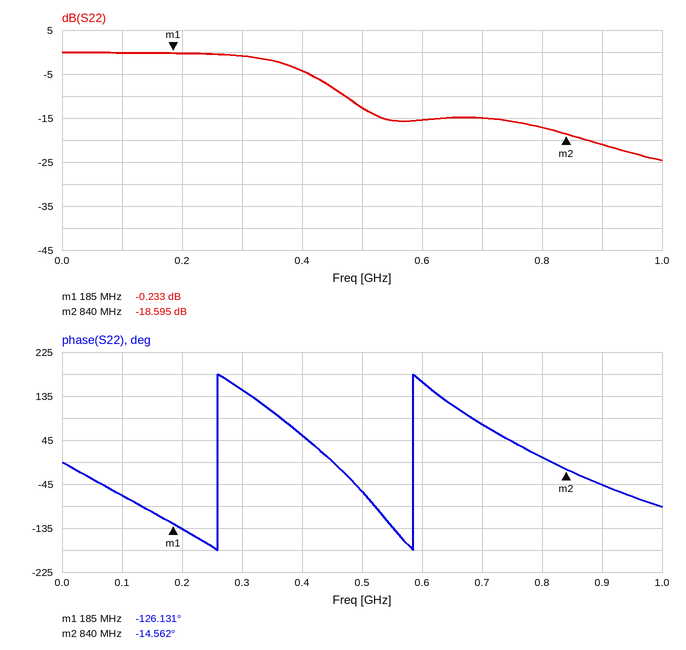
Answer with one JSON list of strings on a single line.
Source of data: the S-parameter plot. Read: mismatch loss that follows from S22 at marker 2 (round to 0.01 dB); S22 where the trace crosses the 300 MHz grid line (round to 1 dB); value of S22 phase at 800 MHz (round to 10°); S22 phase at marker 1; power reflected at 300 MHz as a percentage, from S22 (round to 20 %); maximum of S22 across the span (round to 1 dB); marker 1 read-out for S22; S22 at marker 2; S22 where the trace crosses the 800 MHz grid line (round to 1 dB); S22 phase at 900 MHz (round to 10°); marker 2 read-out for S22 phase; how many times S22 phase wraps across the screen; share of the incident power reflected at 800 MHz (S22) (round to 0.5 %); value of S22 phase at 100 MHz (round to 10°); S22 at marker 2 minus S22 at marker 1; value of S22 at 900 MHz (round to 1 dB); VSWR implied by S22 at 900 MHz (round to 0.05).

["0.06 dB", "-1 dB", "10°", "-126.131°", "80 %", "0 dB", "-0.233 dB", "-18.595 dB", "-17 dB", "-50°", "-14.562°", "2", "2.0 %", "-70°", "-18.362 dB", "-21 dB", "1.20"]
